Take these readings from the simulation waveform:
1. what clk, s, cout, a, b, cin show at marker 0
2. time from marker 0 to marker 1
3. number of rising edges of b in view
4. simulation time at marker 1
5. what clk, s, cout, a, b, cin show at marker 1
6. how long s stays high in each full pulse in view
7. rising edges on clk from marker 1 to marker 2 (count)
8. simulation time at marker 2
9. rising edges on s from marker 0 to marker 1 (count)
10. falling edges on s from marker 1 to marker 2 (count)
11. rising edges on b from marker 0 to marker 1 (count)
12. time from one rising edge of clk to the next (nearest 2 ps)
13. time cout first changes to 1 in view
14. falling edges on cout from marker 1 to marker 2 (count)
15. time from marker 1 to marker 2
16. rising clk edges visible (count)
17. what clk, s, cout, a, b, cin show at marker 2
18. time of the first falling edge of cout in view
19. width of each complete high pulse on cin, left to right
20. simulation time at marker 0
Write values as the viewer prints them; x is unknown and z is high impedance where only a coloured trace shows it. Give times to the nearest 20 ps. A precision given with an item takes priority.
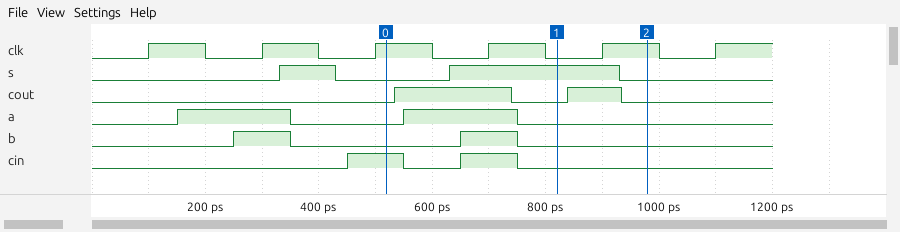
clk=1, s=0, cout=0, a=0, b=0, cin=1
300 ps
2
820 ps
clk=0, s=1, cout=0, a=0, b=0, cin=0
100 ps, 300 ps
1
980 ps
1
1
1
200 ps
540 ps
1
160 ps
6
clk=1, s=0, cout=0, a=0, b=0, cin=0
740 ps
100 ps, 100 ps
520 ps
